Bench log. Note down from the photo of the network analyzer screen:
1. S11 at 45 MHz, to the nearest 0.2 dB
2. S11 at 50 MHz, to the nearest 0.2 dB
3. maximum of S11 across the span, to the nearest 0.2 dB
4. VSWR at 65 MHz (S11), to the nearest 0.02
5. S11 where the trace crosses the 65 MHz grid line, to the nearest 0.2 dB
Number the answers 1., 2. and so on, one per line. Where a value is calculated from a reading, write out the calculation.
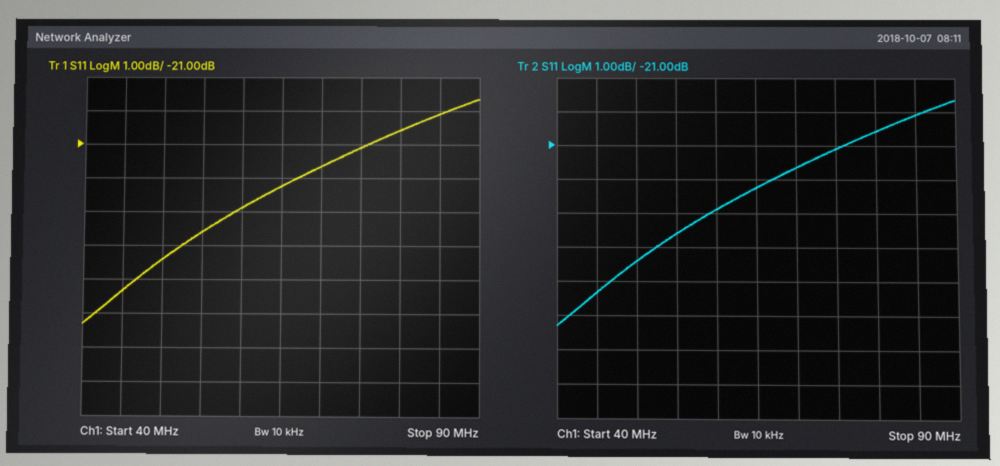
1. -25.4 dB
2. -24.4 dB
3. -19.6 dB
4. |Γ| = 10^(-22.2/20) = 0.0776; VSWR = (1 + 0.0776)/(1 − 0.0776) ≈ 1.17, so 1.16 to the nearest 0.02
5. -22.2 dB
